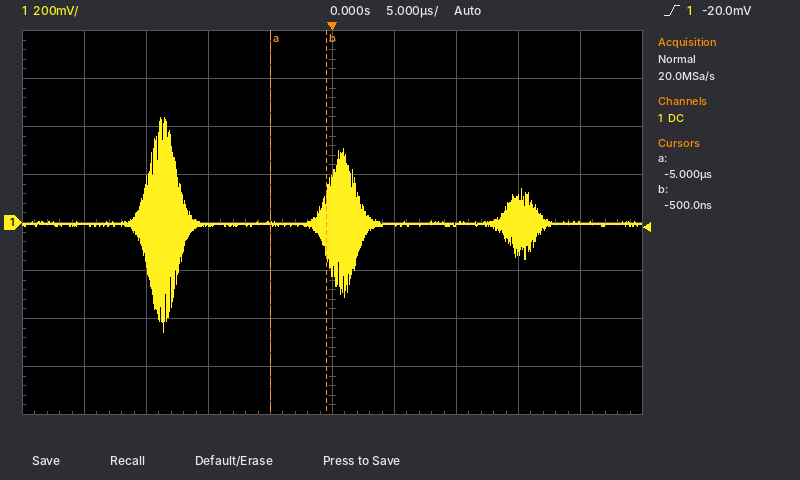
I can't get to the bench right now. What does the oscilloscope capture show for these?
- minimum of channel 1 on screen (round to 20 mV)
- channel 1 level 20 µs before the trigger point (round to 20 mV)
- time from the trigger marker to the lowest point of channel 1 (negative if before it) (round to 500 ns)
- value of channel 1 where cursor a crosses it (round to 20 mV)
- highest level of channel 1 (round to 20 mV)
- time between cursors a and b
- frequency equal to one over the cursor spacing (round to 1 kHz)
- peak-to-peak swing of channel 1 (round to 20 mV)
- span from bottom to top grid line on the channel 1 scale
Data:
-460 mV
0 mV
-13.5 µs
0 mV
440 mV
4.5 µs
222 kHz
900 mV
1.6 V
